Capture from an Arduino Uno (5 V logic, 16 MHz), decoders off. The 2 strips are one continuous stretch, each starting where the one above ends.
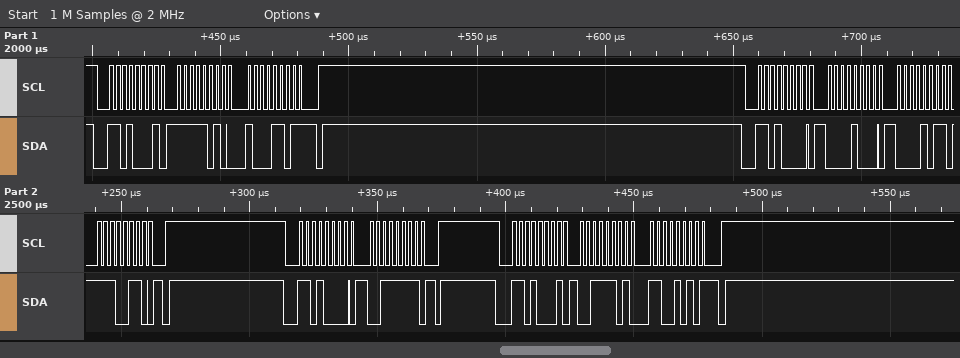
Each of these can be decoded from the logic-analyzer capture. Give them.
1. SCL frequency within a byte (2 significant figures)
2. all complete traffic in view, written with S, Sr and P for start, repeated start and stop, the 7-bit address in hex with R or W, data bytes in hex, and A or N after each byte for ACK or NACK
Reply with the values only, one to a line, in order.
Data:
400 kHz
S 68R A FA A 8D N P S 68W A 08 A 0B A E6 A P S 68W A 3F A P S 68R A 3D A CA N P
